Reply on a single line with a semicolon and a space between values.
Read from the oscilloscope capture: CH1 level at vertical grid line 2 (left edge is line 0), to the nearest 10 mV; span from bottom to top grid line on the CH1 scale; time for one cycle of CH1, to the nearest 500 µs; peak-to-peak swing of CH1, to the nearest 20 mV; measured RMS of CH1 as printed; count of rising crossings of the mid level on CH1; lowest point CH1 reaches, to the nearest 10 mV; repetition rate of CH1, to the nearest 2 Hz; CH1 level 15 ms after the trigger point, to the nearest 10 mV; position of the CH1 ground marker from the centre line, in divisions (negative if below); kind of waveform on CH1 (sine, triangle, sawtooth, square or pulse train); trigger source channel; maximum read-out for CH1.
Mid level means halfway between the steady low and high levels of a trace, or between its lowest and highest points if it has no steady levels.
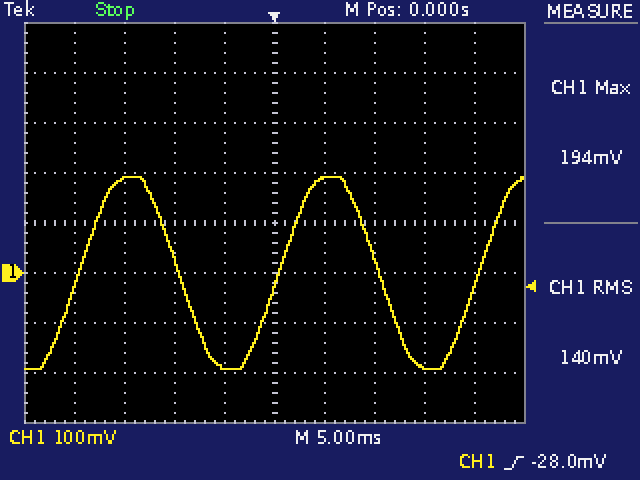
190 mV; 800 mV; 20.0 ms; 380 mV; 140 mV; 3; -190 mV; 50 Hz; -190 mV; -1.0 div; sine; CH1; 194 mV
